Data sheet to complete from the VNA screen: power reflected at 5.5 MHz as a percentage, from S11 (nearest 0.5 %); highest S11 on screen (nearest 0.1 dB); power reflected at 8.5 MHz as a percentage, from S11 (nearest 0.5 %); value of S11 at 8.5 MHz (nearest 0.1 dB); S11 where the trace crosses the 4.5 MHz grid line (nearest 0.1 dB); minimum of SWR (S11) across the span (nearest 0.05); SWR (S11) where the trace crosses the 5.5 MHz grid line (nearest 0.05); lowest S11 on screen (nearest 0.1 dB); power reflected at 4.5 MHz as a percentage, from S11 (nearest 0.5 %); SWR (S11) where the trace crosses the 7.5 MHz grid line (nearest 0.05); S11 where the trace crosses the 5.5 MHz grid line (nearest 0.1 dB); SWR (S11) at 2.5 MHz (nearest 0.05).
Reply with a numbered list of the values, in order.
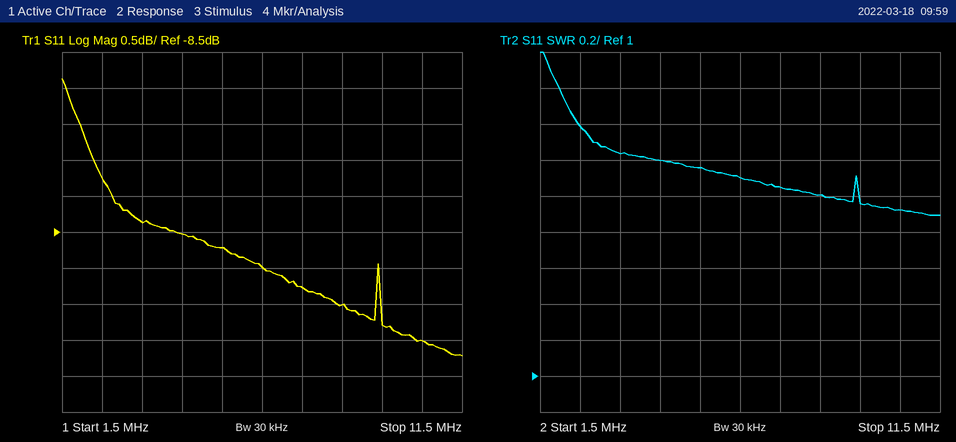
1. 13.5 %
2. -6.4 dB
3. 11.0 %
4. -9.5 dB
5. -8.5 dB
6. 1.90
7. 2.15
8. -10.2 dB
9. 14.0 %
10. 2.05
11. -8.7 dB
12. 2.40
